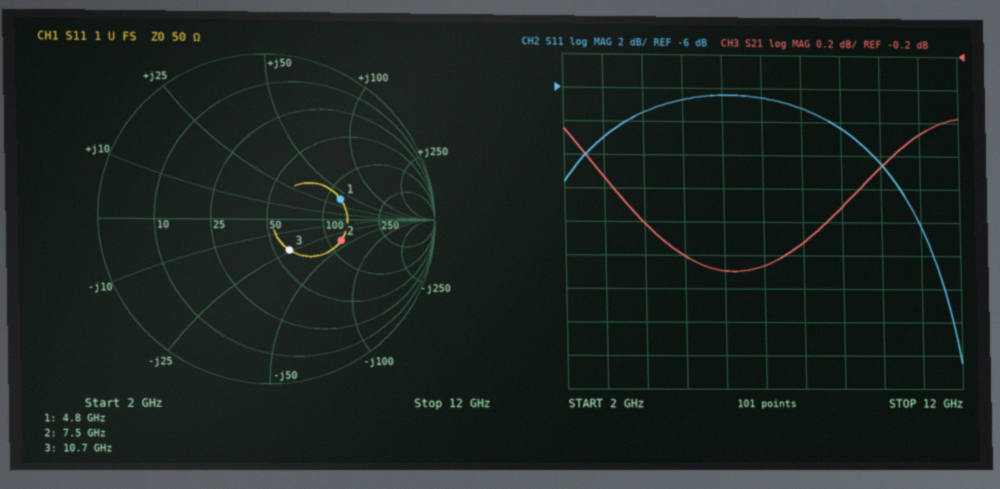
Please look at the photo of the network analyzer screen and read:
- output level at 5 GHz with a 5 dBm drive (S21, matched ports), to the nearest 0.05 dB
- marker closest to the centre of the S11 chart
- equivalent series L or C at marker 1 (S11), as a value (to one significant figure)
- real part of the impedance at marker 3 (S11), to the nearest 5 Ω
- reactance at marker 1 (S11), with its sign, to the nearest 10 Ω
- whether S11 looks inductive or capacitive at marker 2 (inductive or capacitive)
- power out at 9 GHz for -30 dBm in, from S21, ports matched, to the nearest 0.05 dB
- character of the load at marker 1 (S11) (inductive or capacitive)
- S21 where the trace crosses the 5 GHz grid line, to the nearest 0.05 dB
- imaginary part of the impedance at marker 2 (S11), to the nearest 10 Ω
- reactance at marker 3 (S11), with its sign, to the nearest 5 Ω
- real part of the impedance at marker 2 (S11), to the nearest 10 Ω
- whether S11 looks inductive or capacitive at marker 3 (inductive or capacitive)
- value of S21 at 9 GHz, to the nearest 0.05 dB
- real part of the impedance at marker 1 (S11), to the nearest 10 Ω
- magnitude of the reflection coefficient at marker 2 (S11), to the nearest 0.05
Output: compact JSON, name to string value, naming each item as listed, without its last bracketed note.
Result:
{"output level at 5 GHz with a 5 dBm drive (S21, matched ports), to the nearest 0.05 dB": "3.60 dBm", "marker closest to the centre of the S11 chart": "marker 3", "equivalent series L or C at marker 1 (S11), as a value": "1 nH", "real part of the impedance at marker 3 (S11), to the nearest 5 Ω": "60 Ω", "reactance at marker 1 (S11), with its sign, to the nearest 10 Ω": "+40 Ω", "whether S11 looks inductive or capacitive at marker 2": "capacitive", "power out at 9 GHz for -30 dBm in, from S21, ports matched, to the nearest 0.05 dB": "-31.10 dBm", "character of the load at marker 1 (S11)": "inductive", "S21 where the trace crosses the 5 GHz grid line, to the nearest 0.05 dB": "-1.40 dB", "imaginary part of the impedance at marker 2 (S11), to the nearest 10 Ω": "-40 Ω", "reactance at marker 3 (S11), with its sign, to the nearest 5 Ω": "-25 Ω", "real part of the impedance at marker 2 (S11), to the nearest 10 Ω": "120 Ω", "whether S11 looks inductive or capacitive at marker 3": "capacitive", "value of S21 at 9 GHz, to the nearest 0.05 dB": "-1.10 dB", "real part of the impedance at marker 1 (S11), to the nearest 10 Ω": "120 Ω", "magnitude of the reflection coefficient at marker 2 (S11), to the nearest 0.05": "0.45"}
